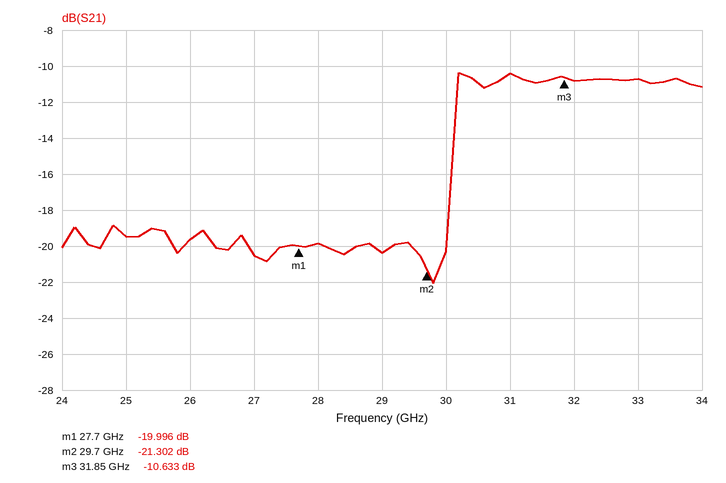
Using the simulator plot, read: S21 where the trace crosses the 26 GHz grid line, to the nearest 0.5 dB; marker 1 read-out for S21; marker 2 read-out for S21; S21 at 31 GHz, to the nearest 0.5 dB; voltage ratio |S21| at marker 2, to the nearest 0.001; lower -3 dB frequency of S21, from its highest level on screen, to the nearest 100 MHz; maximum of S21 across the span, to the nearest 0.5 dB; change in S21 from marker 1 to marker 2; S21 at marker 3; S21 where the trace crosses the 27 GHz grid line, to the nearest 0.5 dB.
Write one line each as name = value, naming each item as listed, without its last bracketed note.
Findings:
S21 where the trace crosses the 26 GHz grid line, to the nearest 0.5 dB = -19.5 dB
marker 1 read-out for S21 = -19.996 dB
marker 2 read-out for S21 = -21.302 dB
S21 at 31 GHz, to the nearest 0.5 dB = -10.5 dB
voltage ratio |S21| at marker 2, to the nearest 0.001 = 0.086
lower -3 dB frequency of S21, from its highest level on screen, to the nearest 100 MHz = 30.1 GHz
maximum of S21 across the span, to the nearest 0.5 dB = -10.5 dB
change in S21 from marker 1 to marker 2 = -1.306 dB
S21 at marker 3 = -10.633 dB
S21 where the trace crosses the 27 GHz grid line, to the nearest 0.5 dB = -20.5 dB
